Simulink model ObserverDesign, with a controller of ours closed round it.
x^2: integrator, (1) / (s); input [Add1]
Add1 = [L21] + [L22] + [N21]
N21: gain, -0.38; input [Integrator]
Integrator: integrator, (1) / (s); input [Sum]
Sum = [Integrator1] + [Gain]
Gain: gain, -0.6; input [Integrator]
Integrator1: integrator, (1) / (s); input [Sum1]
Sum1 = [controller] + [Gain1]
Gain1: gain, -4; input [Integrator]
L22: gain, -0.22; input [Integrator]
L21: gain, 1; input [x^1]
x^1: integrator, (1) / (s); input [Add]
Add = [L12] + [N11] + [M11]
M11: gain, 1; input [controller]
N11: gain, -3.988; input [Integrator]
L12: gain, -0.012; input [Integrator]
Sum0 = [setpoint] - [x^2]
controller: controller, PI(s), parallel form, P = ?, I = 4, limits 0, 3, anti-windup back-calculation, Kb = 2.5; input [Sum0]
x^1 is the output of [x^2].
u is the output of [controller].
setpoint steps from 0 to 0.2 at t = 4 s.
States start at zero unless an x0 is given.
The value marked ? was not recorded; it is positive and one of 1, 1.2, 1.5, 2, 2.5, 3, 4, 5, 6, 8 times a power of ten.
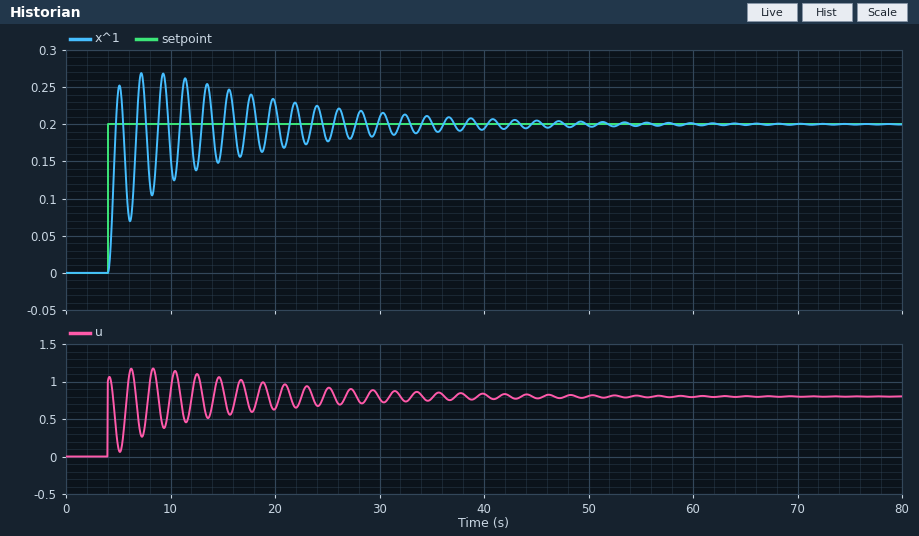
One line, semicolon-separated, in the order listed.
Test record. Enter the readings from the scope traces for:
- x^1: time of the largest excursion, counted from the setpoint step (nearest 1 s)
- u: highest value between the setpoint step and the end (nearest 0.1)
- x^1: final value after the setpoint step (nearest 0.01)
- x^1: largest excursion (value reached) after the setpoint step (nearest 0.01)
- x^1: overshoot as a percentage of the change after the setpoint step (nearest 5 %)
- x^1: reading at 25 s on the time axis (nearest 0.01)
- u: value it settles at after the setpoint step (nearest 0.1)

3 s; 1.2; 0.20; 0.27; 35 %; 0.18; 0.8
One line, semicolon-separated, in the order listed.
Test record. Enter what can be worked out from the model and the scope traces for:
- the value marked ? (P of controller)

5
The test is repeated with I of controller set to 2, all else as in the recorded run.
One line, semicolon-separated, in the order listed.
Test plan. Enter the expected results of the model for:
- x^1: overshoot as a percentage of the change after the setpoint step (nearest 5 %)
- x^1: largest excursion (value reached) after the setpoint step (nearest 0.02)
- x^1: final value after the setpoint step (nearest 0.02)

10 %; 0.22; 0.20
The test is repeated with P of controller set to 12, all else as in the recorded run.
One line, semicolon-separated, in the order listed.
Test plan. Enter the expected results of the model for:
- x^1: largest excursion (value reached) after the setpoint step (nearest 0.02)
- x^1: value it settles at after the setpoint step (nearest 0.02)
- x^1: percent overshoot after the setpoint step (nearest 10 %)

0.32; 0.20; 60 %
